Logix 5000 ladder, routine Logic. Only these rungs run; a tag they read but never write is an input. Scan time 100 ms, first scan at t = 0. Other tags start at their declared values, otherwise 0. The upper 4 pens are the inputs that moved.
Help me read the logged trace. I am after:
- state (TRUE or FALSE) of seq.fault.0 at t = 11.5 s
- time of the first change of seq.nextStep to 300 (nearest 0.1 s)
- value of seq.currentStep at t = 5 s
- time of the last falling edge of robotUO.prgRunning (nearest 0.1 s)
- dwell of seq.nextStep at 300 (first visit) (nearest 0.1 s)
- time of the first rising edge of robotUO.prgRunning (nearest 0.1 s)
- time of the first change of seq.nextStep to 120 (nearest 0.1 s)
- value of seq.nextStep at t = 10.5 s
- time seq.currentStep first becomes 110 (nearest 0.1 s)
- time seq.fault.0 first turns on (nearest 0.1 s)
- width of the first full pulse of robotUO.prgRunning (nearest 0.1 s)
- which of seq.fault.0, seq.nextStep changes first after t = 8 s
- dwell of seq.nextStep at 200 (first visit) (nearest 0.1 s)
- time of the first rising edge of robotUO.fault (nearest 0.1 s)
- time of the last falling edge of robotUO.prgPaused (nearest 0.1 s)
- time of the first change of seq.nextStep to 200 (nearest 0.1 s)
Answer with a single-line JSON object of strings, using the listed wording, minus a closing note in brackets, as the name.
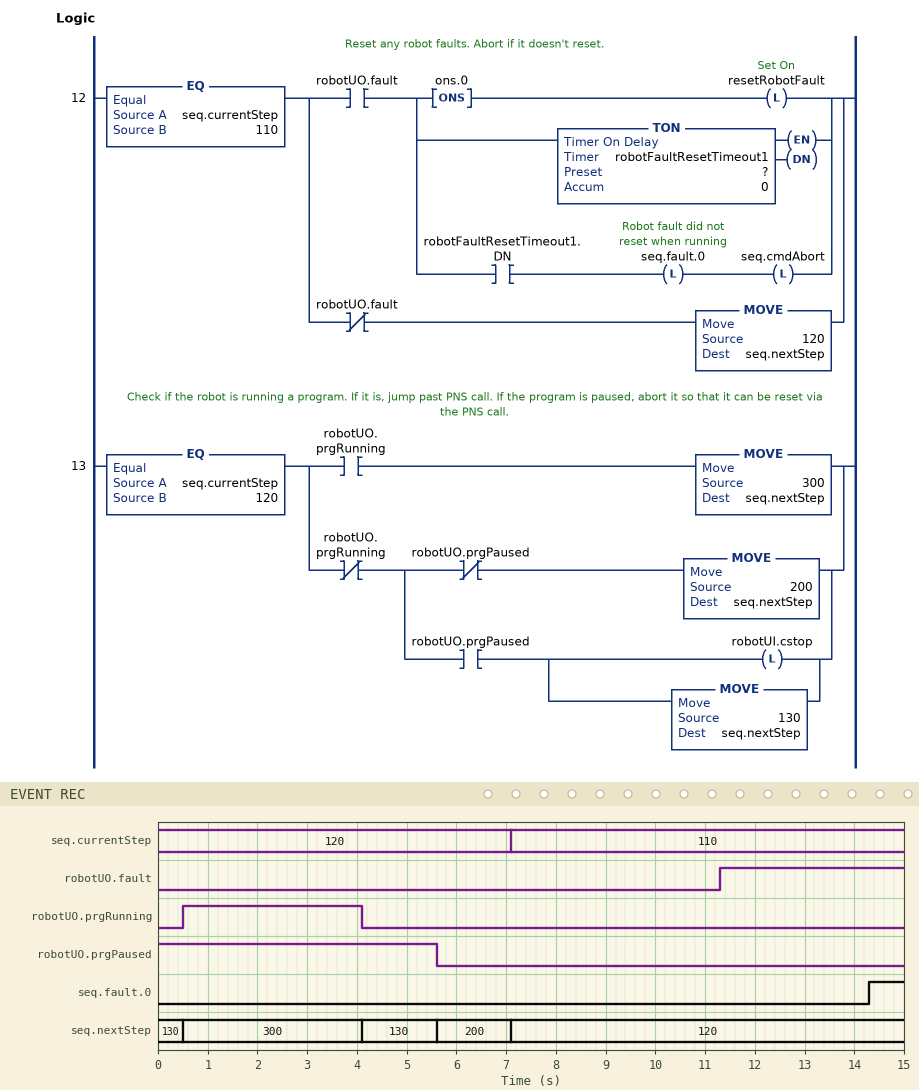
{"state (TRUE or FALSE) of seq.fault.0 at t = 11.5 s": "FALSE", "time of the first change of seq.nextStep to 300": "0.5 s", "value of seq.currentStep at t = 5 s": "120", "time of the last falling edge of robotUO.prgRunning": "4.1 s", "dwell of seq.nextStep at 300 (first visit)": "3.6 s", "time of the first rising edge of robotUO.prgRunning": "0.5 s", "time of the first change of seq.nextStep to 120": "7.1 s", "value of seq.nextStep at t = 10.5 s": "120", "time seq.currentStep first becomes 110": "7.1 s", "time seq.fault.0 first turns on": "14.3 s", "width of the first full pulse of robotUO.prgRunning": "3.6 s", "which of seq.fault.0, seq.nextStep changes first after t = 8 s": "seq.fault.0", "dwell of seq.nextStep at 200 (first visit)": "1.5 s", "time of the first rising edge of robotUO.fault": "11.3 s", "time of the last falling edge of robotUO.prgPaused": "5.6 s", "time of the first change of seq.nextStep to 200": "5.6 s"}
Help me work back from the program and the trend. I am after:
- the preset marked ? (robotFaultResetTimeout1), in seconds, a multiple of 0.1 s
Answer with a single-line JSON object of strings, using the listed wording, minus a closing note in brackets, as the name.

{"the preset marked ? (robotFaultResetTimeout1), in seconds, a multiple of 0.1 s": "3.0 s"}
